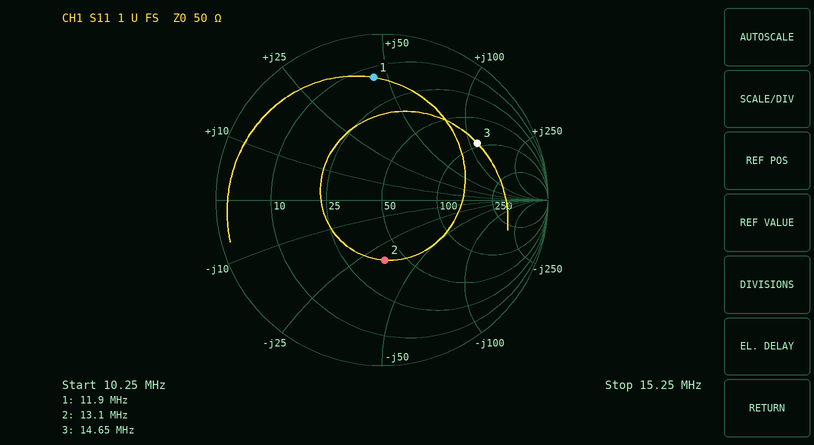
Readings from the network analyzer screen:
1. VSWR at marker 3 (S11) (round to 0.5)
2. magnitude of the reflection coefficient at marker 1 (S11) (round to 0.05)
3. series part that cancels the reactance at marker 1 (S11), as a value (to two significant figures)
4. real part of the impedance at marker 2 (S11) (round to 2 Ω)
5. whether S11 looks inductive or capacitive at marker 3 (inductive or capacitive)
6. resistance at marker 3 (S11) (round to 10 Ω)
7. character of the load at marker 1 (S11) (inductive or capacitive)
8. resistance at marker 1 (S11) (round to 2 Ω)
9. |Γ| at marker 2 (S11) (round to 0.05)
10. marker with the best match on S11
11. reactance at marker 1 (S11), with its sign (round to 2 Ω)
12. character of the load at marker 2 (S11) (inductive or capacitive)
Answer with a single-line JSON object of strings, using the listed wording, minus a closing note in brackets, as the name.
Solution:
{"VSWR at marker 3 (S11)": "5.0", "magnitude of the reflection coefficient at marker 1 (S11)": "0.75", "series part that cancels the reactance at marker 1 (S11), as a value": "300 pF", "real part of the impedance at marker 2 (S11)": "40 Ω", "whether S11 looks inductive or capacitive at marker 3": "inductive", "resistance at marker 3 (S11)": "90 Ω", "character of the load at marker 1 (S11)": "inductive", "resistance at marker 1 (S11)": "14 Ω", "|Γ| at marker 2 (S11)": "0.35", "marker with the best match on S11": "marker 2", "reactance at marker 1 (S11), with its sign": "+44 Ω", "character of the load at marker 2 (S11)": "capacitive"}
